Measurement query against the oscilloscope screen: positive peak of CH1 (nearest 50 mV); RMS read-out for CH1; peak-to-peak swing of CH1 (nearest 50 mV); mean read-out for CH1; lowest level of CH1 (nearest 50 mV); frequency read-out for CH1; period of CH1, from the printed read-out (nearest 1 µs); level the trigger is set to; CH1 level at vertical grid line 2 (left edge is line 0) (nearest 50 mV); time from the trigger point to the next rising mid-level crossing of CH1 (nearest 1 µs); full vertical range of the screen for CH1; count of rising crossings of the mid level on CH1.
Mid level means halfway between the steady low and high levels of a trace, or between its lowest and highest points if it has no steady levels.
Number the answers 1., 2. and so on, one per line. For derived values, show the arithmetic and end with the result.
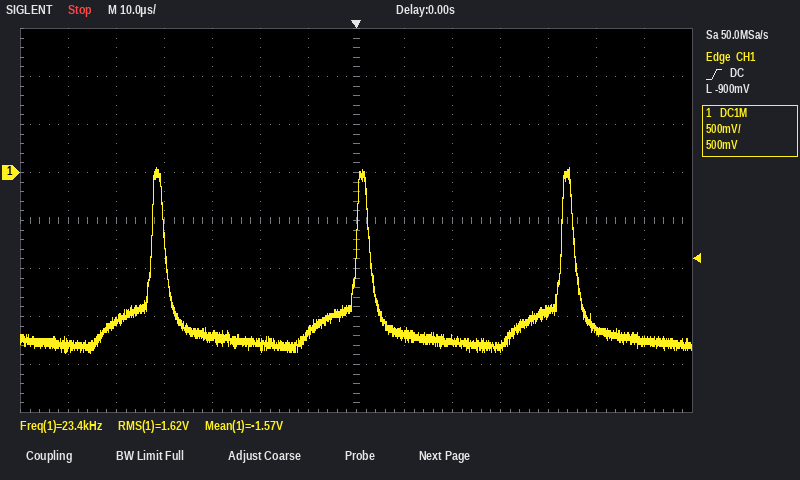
1. 50 mV
2. 1.62 V
3. 50 mV − (-1.90 V) = 1.95 V
4. -1.57 V
5. -1.90 V
6. 23.4 kHz
7. 1 / 23.4 kHz ≈ 43 µs
8. -900 mV
9. -1.55 V
10. 43 µs
11. 4 V
12. 3
